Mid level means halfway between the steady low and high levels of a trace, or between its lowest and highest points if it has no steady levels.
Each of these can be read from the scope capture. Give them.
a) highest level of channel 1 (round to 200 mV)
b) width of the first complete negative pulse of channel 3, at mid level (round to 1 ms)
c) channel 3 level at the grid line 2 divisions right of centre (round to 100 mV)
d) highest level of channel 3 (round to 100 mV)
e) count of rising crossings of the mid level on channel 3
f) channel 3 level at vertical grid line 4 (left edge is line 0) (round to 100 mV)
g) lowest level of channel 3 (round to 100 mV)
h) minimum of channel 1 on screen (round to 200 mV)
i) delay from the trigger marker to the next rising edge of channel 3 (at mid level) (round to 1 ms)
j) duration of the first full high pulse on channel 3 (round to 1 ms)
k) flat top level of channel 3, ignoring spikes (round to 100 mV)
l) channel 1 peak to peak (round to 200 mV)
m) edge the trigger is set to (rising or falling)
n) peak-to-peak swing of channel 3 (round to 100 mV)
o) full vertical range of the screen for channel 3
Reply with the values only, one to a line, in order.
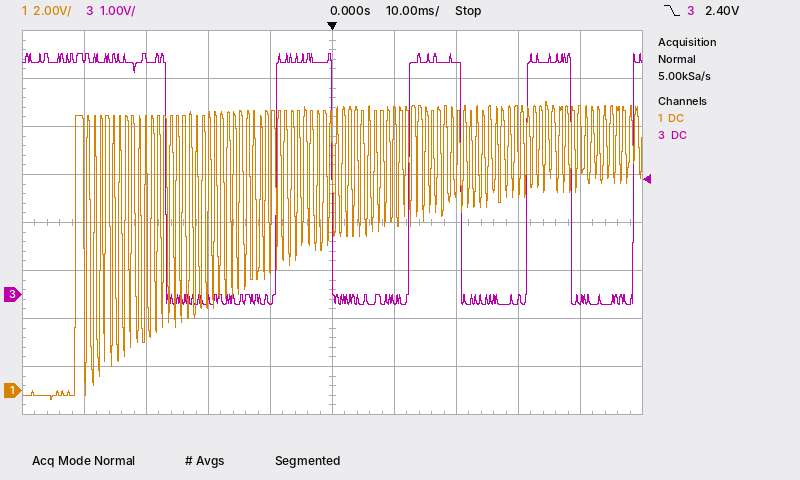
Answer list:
12.0 V
18 ms
4.8 V
5.0 V
4
-100 mV
-200 mV
-400 mV
12 ms
9 ms
4.8 V
12.4 V
falling
5.2 V
8 V
